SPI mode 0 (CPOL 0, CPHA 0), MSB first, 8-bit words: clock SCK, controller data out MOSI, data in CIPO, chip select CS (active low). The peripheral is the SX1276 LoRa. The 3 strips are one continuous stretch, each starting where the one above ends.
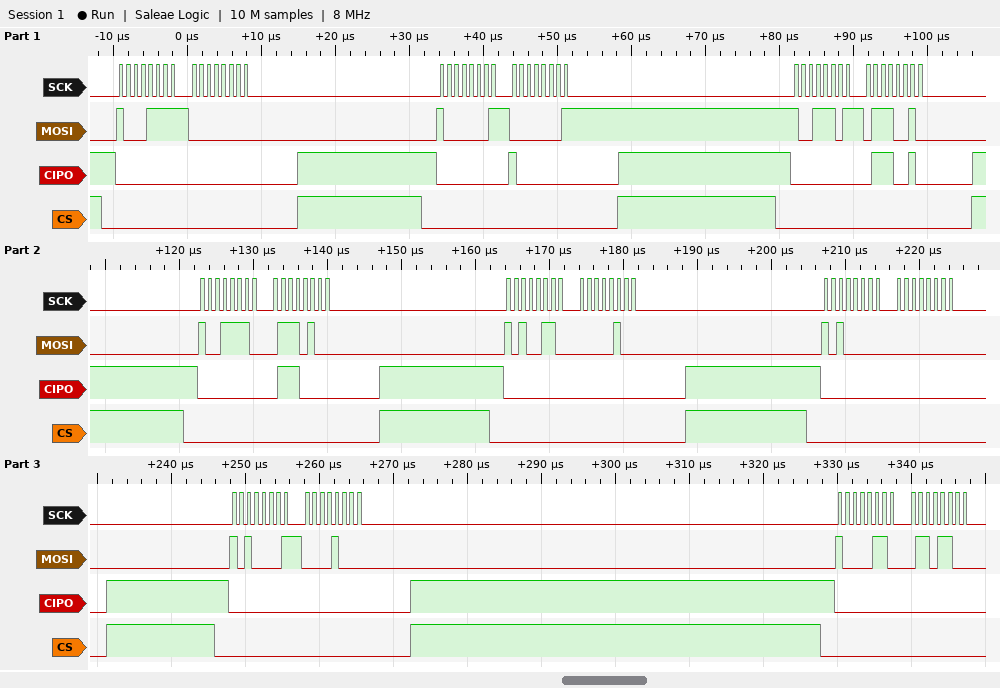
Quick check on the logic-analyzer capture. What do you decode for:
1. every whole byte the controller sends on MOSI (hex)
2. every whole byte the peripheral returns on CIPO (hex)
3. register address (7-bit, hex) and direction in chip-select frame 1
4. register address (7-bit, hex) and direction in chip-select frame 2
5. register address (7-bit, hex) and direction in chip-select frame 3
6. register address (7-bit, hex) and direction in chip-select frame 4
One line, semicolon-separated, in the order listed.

8F 00 81 01 9D 72 9E 74 A6 04 A0 00 A1 08 86 6C; 00 00 00 80 00 72 00 70 00 00 00 00 00 00 00 00; 0x0F write; 0x01 write; 0x1D write; 0x1E write
